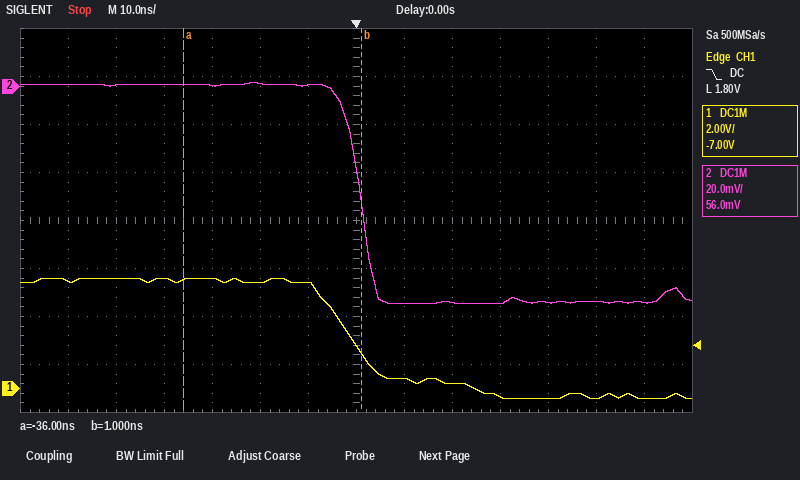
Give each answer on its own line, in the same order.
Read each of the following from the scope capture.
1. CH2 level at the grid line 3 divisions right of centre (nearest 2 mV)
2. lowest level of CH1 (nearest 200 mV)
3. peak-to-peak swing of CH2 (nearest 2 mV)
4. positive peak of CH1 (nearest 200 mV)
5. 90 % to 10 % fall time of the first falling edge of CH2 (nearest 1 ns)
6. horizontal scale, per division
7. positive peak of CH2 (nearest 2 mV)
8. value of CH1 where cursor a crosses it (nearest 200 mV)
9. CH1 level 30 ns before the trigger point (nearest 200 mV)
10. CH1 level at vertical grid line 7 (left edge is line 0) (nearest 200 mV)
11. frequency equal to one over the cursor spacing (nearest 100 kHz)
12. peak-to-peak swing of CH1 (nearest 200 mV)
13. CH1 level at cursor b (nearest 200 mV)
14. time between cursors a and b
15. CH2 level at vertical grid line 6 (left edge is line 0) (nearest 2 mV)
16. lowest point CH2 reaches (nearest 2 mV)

-90 mV
-400 mV
92 mV
4.6 V
7 ns
10 ns
2 mV
4.6 V
4.6 V
1.8 V
27.0 MHz
5.0 V
1.4 V
37 ns
0 mV
-90 mV
